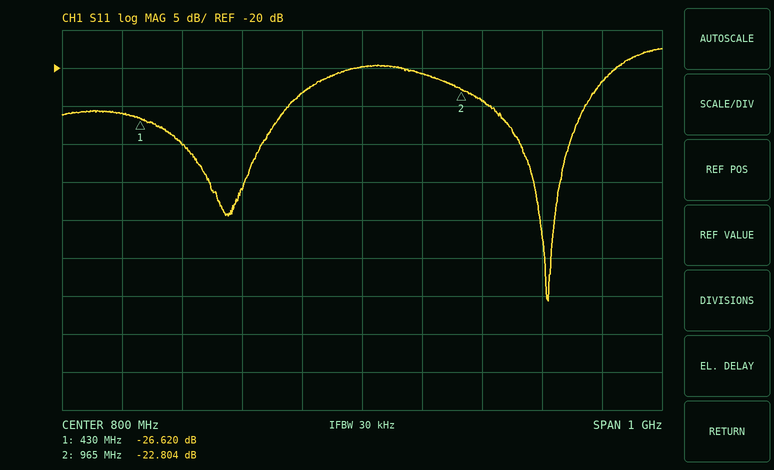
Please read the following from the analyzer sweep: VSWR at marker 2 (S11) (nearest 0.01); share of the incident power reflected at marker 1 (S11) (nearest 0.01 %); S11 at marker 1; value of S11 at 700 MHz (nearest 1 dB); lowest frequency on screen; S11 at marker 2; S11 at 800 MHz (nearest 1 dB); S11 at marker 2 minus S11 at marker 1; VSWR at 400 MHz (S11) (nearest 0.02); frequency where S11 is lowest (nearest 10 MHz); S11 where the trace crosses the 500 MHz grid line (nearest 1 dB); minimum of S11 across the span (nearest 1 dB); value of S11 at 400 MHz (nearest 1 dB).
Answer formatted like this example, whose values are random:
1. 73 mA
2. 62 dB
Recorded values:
1. 1.16
2. 0.22 %
3. -26.620 dB
4. -23 dB
5. 300 MHz
6. -22.804 dB
7. -20 dB
8. 3.816 dB
9. 1.10
10. 1.11 GHz
11. -30 dB
12. -51 dB
13. -26 dB
